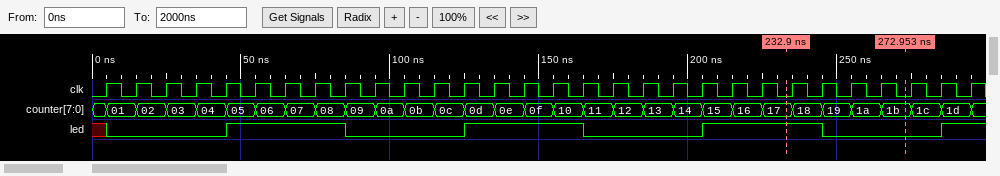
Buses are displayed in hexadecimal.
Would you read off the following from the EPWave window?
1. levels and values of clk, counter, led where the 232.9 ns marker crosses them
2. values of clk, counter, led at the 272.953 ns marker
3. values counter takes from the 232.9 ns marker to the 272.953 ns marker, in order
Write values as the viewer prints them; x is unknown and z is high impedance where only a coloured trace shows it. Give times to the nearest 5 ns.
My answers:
clk=0, counter=17, led=1
clk=0, counter=1b, led=0
17, 18, 19, 1a, 1b
